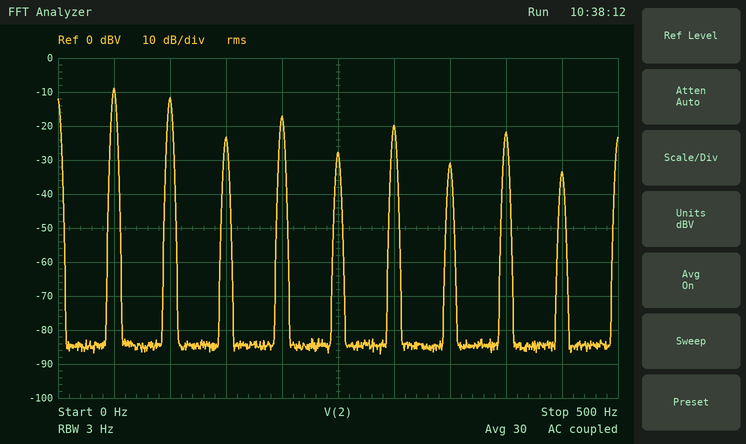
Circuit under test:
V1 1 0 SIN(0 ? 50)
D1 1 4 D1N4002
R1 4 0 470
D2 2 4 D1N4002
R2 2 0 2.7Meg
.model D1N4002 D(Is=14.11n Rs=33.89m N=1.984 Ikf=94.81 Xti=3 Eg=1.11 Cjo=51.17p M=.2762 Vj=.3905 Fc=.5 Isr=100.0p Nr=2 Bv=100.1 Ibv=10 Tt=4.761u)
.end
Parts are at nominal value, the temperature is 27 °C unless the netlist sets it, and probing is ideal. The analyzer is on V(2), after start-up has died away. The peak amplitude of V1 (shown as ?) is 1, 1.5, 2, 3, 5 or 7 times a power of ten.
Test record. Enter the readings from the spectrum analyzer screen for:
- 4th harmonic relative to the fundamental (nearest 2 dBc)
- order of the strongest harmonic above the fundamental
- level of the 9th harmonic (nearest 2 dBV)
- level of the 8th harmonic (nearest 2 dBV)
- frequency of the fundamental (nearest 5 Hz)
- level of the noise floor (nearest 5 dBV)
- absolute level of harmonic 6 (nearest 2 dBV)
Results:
-8 dBc
2
-34 dBV
-22 dBV
50 Hz
-85 dBV
-20 dBV
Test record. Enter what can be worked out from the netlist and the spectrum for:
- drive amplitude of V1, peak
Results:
70 V
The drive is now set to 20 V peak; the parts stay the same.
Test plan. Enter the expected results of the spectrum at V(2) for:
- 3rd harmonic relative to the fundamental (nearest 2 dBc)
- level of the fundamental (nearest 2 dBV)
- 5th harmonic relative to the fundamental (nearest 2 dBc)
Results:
-16 dBc
-18 dBV
-24 dBc
